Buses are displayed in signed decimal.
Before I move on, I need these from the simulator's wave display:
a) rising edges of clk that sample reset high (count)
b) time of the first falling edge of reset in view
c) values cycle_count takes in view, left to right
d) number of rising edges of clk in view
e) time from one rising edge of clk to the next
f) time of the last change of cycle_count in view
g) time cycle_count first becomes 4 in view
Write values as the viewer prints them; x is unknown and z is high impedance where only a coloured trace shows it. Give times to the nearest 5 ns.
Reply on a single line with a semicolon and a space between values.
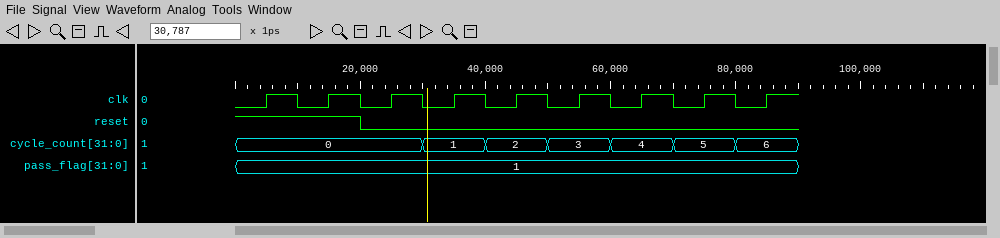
2; 20 ns; 0, 1, 2, 3, 4, 5, 6; 9; 10 ns; 80 ns; 60 ns
